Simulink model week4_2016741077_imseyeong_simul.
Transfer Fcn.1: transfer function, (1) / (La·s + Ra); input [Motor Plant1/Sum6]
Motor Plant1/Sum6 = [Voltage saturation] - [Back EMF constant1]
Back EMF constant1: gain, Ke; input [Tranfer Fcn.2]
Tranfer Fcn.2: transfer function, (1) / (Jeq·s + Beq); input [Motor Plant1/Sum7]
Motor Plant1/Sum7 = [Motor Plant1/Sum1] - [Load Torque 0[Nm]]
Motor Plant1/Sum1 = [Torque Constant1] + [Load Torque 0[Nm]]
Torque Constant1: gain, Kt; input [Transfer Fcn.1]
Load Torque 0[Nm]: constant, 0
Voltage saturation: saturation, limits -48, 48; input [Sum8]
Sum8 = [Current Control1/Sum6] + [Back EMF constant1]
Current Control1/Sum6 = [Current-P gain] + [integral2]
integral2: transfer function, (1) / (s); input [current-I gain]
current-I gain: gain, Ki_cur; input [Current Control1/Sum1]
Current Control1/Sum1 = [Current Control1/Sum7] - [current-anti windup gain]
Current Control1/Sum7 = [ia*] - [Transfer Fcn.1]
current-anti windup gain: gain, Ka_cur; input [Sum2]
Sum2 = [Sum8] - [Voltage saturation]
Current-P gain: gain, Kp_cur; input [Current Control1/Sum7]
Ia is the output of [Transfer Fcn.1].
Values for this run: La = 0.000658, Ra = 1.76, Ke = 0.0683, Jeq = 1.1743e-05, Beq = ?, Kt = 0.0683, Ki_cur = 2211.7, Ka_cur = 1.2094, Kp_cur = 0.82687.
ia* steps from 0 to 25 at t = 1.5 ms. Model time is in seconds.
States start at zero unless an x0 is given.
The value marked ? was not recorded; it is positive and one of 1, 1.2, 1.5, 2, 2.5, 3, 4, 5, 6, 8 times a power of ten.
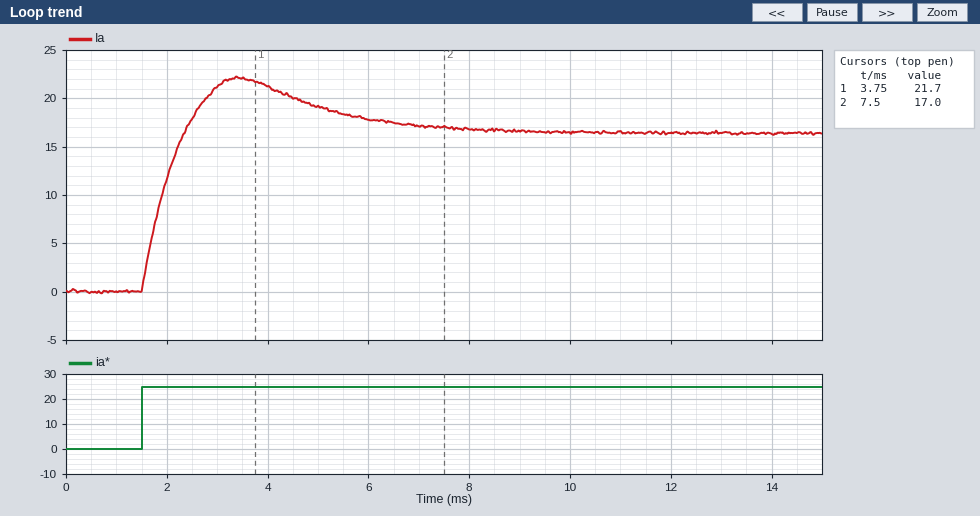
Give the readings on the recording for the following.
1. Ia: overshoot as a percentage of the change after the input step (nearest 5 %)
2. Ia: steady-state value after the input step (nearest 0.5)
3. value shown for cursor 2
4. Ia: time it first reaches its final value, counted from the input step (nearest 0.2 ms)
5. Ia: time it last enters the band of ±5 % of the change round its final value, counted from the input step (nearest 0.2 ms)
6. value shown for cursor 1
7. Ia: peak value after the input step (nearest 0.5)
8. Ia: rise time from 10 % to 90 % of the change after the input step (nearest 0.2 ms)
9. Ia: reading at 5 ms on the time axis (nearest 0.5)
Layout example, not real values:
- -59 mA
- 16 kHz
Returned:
- 35 %
- 16.5
- 17.0
- 0.8 ms
- 5.4 ms
- 21.7
- 22.0
- 0.6 ms
- 19.0
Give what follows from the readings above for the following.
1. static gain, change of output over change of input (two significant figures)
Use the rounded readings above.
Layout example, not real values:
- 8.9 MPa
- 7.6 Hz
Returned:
- 0.66
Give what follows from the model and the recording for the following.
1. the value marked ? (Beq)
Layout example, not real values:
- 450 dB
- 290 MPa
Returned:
- 0.004
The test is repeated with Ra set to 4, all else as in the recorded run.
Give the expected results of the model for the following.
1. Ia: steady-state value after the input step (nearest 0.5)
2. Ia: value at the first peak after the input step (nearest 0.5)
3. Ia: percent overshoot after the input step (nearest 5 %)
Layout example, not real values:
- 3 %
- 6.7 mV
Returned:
- 9.5
- 11.0
- 20 %
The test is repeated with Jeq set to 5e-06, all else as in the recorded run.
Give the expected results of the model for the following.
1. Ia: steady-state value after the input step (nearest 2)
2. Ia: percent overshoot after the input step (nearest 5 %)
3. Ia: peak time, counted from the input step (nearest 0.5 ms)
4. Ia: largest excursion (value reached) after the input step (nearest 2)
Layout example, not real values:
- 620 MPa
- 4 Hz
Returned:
- 16
- 25 %
- 1.5 ms
- 20
